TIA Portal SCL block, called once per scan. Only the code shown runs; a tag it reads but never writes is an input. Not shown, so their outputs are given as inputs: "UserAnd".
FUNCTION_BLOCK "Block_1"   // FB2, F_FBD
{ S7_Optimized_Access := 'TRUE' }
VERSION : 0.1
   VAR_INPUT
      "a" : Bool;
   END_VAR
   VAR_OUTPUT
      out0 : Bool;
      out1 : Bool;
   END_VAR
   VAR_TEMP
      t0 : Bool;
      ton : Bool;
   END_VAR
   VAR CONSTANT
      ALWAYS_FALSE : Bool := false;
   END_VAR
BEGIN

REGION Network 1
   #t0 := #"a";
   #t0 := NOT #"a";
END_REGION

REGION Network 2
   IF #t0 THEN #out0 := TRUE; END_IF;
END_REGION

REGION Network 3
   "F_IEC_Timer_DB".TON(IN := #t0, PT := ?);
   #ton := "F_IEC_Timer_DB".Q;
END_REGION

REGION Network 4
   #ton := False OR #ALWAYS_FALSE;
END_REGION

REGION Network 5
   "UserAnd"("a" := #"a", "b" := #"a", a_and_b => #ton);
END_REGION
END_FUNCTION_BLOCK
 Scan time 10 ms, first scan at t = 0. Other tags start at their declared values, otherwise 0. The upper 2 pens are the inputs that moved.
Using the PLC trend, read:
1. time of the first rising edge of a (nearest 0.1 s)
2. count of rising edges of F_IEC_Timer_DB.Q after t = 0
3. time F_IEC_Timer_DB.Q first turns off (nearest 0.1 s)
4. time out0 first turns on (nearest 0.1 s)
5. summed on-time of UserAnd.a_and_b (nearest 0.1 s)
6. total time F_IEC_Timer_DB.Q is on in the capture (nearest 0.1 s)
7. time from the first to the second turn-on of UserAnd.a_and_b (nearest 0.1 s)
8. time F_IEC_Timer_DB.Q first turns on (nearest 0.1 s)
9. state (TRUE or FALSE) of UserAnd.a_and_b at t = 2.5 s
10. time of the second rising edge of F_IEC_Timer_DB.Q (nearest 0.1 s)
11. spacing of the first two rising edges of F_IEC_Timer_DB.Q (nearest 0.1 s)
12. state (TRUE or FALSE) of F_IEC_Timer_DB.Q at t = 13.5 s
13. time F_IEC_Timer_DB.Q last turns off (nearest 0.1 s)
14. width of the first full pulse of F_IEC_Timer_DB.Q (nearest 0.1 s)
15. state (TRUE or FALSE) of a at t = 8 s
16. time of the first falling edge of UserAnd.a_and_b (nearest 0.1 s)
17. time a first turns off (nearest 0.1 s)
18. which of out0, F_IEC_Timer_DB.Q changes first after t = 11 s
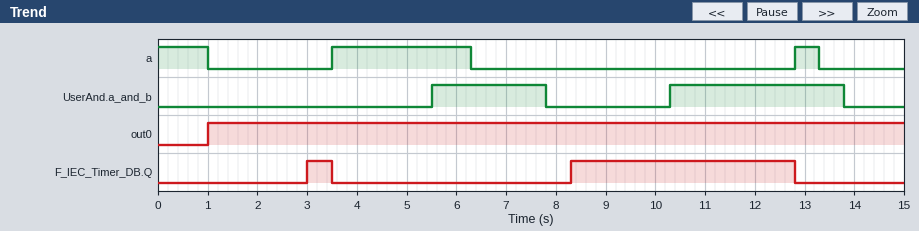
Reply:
3.5 s
2
3.5 s
1.0 s
5.8 s
5.0 s
4.8 s
3.0 s
FALSE
8.3 s
5.3 s
FALSE
12.8 s
0.5 s
FALSE
7.8 s
1.0 s
F_IEC_Timer_DB.Q
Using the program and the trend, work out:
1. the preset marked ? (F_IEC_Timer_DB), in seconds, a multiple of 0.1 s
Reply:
2.0 s
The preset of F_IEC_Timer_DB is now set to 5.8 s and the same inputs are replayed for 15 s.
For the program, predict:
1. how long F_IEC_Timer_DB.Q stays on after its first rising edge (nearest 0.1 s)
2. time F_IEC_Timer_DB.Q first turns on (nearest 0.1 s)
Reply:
0.7 s
12.1 s
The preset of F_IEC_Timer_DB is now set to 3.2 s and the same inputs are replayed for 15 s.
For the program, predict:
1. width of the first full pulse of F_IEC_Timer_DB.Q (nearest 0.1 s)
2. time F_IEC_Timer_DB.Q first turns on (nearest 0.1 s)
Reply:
3.3 s
9.5 s
